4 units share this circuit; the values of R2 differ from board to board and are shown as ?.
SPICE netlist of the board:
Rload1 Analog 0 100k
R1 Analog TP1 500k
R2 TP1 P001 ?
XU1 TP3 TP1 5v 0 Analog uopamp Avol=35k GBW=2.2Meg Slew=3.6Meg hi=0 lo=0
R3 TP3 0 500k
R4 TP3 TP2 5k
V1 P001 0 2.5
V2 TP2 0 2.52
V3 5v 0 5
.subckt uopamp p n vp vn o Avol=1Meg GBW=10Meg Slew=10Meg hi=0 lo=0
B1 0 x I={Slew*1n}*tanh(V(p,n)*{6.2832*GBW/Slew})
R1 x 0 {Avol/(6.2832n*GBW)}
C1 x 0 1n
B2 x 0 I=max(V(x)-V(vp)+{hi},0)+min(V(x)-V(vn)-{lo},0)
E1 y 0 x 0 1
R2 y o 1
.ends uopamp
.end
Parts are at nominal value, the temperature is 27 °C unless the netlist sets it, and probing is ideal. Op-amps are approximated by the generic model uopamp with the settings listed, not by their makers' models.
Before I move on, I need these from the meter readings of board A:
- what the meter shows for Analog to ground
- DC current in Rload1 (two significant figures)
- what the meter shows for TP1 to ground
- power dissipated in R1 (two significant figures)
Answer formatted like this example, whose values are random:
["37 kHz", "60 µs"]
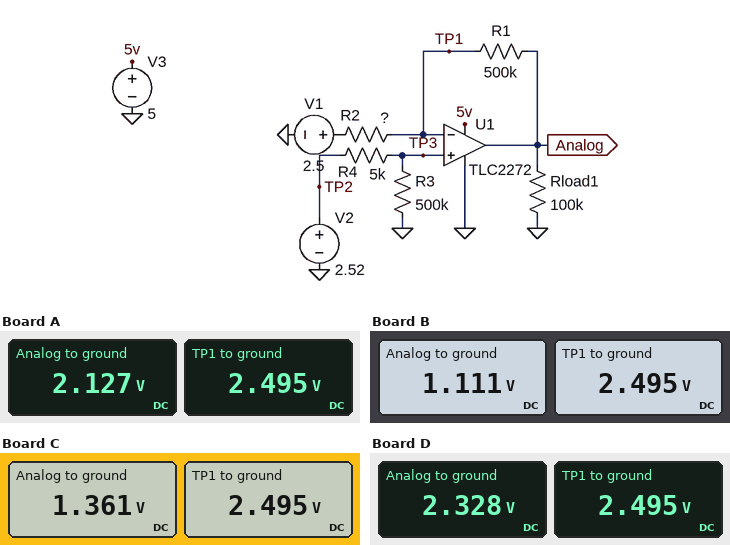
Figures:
["2.127 V", "21 µA", "2.495 V", "270 nW"]
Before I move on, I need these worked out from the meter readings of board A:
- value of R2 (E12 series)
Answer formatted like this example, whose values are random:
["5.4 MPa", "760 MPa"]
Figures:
["6.8 kΩ"]
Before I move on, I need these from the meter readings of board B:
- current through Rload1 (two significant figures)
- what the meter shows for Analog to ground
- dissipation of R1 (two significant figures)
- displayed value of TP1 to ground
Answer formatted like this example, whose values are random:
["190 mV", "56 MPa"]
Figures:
["11 µA", "1.111 V", "3.8 µW", "2.495 V"]
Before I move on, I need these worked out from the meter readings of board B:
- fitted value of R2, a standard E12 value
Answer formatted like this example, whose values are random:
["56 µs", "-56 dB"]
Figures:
["1.8 kΩ"]
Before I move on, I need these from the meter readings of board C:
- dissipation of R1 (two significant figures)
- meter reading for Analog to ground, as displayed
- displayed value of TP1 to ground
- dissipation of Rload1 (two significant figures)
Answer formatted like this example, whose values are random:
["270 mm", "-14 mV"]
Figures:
["2.6 µW", "1.361 V", "2.495 V", "19 µW"]
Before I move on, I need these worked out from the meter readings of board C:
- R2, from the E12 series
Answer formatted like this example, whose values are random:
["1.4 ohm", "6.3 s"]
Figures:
["2.2 kΩ"]
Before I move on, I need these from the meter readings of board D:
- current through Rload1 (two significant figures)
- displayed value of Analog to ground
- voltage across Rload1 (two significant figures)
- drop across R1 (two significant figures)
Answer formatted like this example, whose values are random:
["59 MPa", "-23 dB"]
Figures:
["23 µA", "2.328 V", "2.3 V", "170 mV"]
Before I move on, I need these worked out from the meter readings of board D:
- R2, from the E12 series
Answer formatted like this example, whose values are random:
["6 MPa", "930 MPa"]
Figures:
["15 kΩ"]
